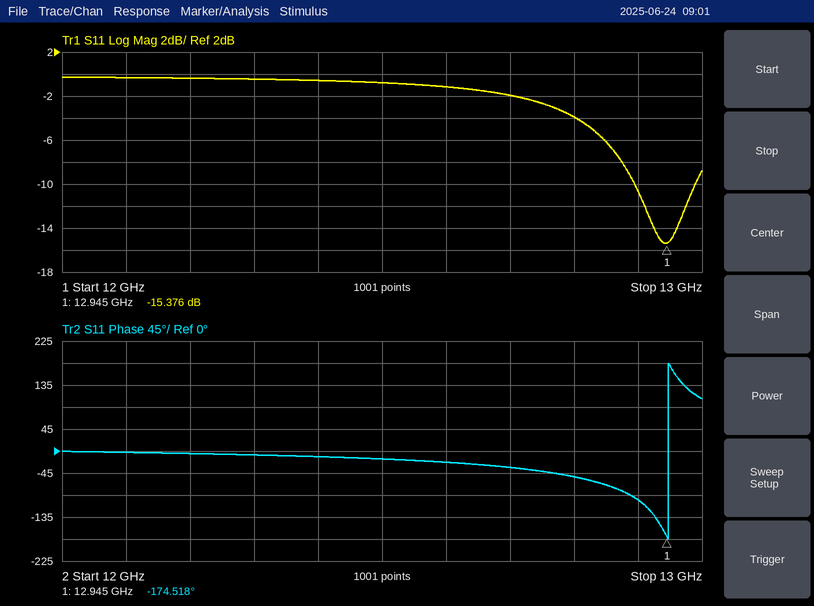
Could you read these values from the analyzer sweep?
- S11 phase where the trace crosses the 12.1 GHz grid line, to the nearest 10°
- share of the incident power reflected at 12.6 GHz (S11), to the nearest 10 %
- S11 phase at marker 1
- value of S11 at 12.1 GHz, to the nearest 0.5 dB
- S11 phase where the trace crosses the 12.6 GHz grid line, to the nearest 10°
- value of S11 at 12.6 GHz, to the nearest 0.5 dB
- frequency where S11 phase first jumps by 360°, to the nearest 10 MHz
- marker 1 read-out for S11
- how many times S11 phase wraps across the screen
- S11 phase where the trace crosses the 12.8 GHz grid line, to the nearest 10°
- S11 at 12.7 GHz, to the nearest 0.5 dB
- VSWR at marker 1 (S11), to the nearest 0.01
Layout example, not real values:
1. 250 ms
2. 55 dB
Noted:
1. 0°
2. 80 %
3. -174.518°
4. -0.5 dB
5. -20°
6. -1.0 dB
7. 12.95 GHz
8. -15.376 dB
9. 1
10. -50°
11. -2.0 dB
12. 1.41
